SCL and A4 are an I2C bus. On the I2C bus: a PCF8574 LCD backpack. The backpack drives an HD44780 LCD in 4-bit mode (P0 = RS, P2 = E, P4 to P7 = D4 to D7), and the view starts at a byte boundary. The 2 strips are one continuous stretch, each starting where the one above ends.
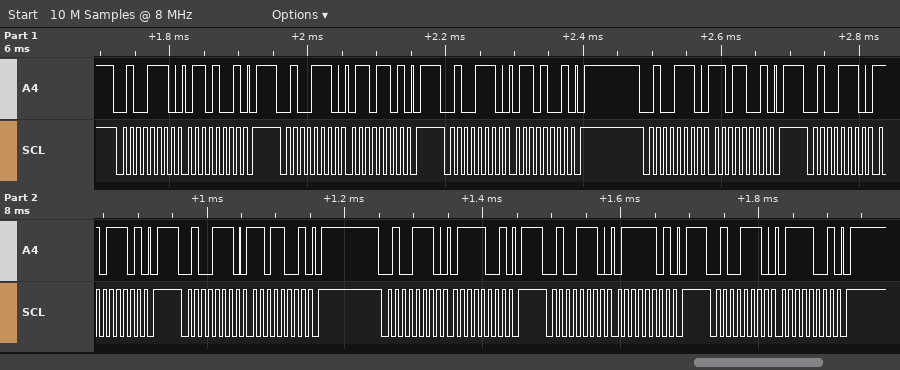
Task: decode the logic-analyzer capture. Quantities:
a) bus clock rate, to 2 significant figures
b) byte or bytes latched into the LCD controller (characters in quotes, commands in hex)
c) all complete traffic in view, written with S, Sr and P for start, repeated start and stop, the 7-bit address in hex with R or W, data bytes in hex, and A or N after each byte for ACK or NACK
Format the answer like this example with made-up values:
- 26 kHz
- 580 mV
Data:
- 100 kHz
- 'm'
- S 27W A 69 A P S 27W A 6D A P S 27W A 69 A P S 27W A D9 A P S 27W A DD A P S 27W A D9 A P S 27W A 79 A P S 27W A 7D A P S 27W A 79 A P
